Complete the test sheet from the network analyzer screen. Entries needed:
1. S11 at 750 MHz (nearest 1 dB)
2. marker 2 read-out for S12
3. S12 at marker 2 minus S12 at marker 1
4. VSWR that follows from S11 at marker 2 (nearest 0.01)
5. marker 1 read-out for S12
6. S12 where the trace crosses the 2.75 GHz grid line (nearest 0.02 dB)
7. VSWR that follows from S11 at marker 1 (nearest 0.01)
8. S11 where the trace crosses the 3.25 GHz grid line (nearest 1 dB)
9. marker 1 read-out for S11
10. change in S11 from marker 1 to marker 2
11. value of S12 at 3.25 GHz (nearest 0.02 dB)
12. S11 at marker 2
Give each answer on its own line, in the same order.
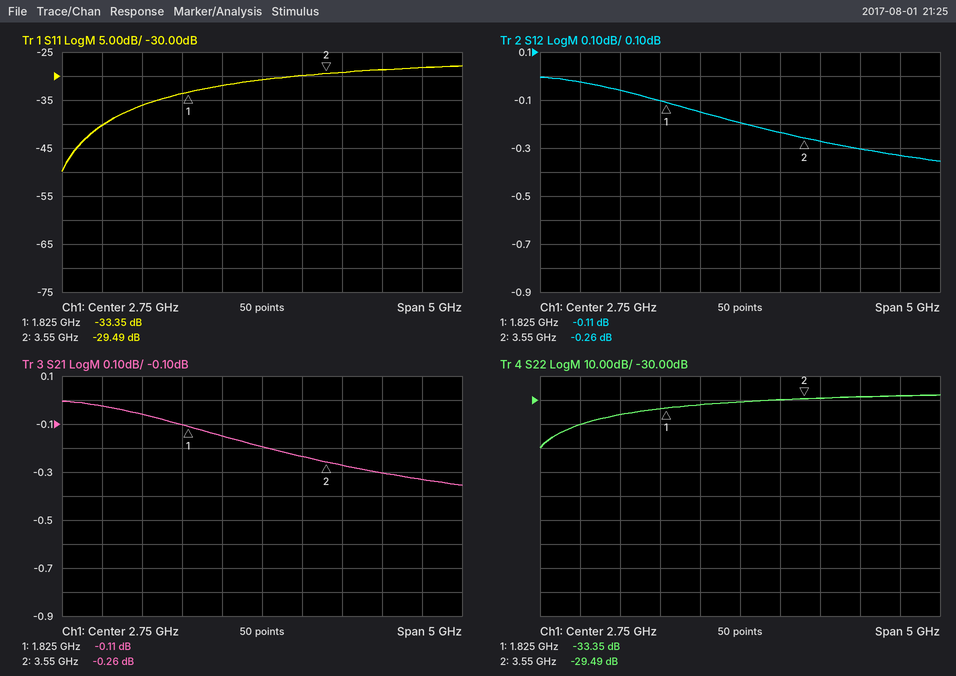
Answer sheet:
-40 dB
-0.26 dB
-0.15 dB
1.07
-0.11 dB
-0.20 dB
1.04
-30 dB
-33.35 dB
3.86 dB
-0.24 dB
-29.49 dB
